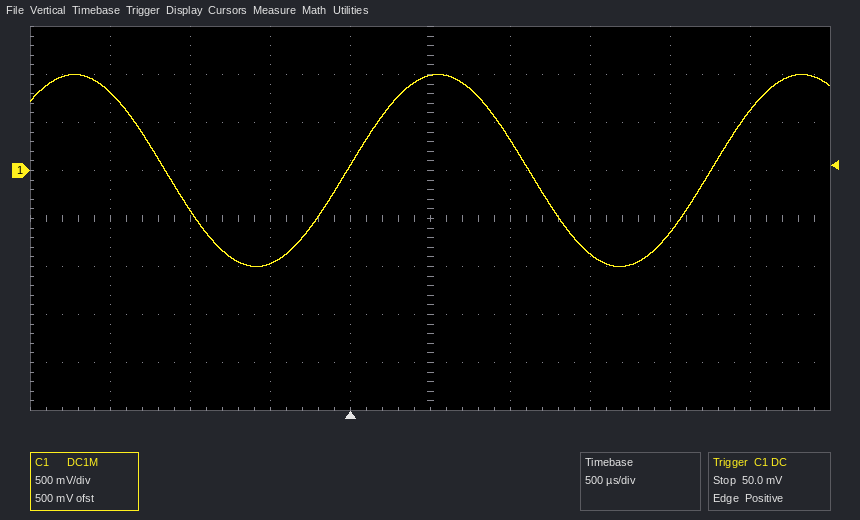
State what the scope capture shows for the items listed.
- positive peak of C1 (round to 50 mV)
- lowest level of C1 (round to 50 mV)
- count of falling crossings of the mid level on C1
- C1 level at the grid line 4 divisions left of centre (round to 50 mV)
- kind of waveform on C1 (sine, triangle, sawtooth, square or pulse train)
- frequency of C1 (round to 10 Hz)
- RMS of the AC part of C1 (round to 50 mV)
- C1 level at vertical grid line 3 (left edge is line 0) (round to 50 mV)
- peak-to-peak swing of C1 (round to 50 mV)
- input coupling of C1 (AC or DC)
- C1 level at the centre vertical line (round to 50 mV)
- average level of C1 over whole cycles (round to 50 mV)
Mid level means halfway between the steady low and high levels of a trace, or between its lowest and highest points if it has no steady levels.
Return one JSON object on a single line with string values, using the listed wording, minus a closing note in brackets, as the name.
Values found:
{"positive peak of C1": "1.00 V", "lowest level of C1": "-1.00 V", "count of falling crossings of the mid level on C1": "2", "C1 level at the grid line 4 divisions left of centre": "800 mV", "kind of waveform on C1": "sine", "frequency of C1": "440 Hz", "RMS of the AC part of C1": "700 mV", "C1 level at vertical grid line 3 (left edge is line 0)": "-950 mV", "peak-to-peak swing of C1": "2.00 V", "input coupling of C1": "DC", "C1 level at the centre vertical line": "1.00 V", "average level of C1 over whole cycles": "0 mV"}
